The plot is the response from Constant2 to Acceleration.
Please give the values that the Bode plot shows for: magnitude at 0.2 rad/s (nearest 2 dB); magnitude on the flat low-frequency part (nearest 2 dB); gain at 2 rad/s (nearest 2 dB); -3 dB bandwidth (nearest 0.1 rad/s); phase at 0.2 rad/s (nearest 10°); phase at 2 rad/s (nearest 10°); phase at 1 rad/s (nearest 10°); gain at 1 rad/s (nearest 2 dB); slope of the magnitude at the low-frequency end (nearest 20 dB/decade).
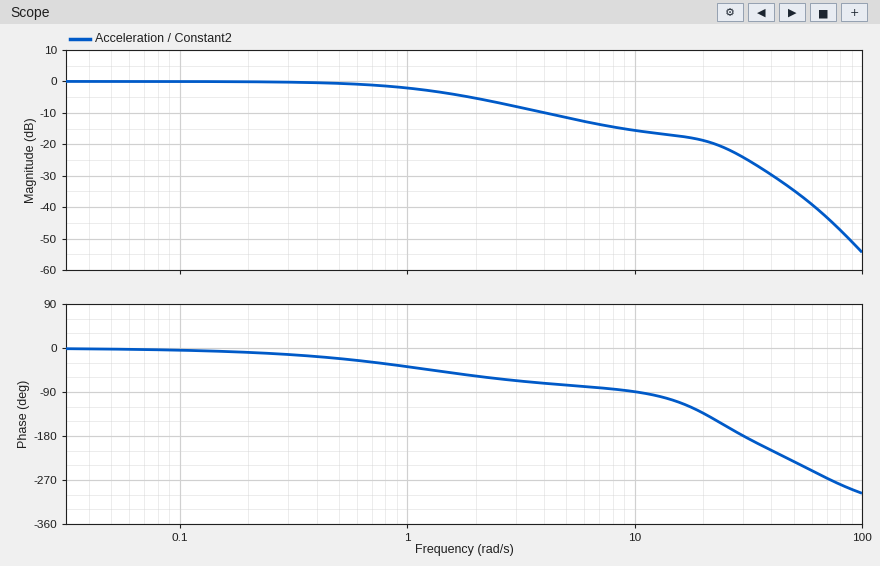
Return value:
0 dB
0 dB
-6 dB
1.3 rad/s
-10°
-60°
-40°
-2 dB
0 dB/decade
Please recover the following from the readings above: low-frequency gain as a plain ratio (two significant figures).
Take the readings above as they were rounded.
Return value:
1.0
